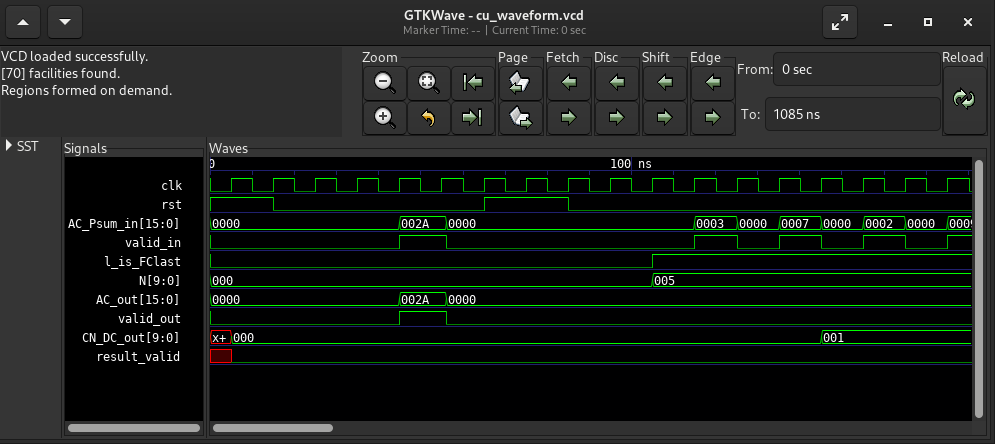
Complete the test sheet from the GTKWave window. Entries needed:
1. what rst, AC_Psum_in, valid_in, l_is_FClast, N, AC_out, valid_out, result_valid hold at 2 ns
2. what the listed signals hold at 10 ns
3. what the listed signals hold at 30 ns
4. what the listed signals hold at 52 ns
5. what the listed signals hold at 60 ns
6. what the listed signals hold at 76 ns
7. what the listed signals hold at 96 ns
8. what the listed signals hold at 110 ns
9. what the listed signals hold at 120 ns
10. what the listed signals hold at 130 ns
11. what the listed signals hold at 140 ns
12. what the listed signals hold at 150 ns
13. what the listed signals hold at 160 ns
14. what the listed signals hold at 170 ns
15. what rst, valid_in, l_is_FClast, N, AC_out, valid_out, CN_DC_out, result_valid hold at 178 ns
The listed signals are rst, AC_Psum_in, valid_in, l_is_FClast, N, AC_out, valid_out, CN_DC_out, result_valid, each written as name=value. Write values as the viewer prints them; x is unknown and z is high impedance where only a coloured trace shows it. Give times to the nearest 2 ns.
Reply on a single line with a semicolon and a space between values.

rst=1, AC_Psum_in=0000, valid_in=0, l_is_FClast=0, N=000, AC_out=0000, valid_out=0, result_valid=x; rst=1, AC_Psum_in=0000, valid_in=0, l_is_FClast=0, N=000, AC_out=0000, valid_out=0, CN_DC_out=000, result_valid=0; rst=0, AC_Psum_in=0000, valid_in=0, l_is_FClast=0, N=000, AC_out=0000, valid_out=0, CN_DC_out=000, result_valid=0; rst=0, AC_Psum_in=002A, valid_in=1, l_is_FClast=0, N=000, AC_out=002A, valid_out=1, CN_DC_out=000, result_valid=0; rst=0, AC_Psum_in=0000, valid_in=0, l_is_FClast=0, N=000, AC_out=0000, valid_out=0, CN_DC_out=000, result_valid=0; rst=1, AC_Psum_in=0000, valid_in=0, l_is_FClast=0, N=000, AC_out=0000, valid_out=0, CN_DC_out=000, result_valid=0; rst=0, AC_Psum_in=0000, valid_in=0, l_is_FClast=0, N=000, AC_out=0000, valid_out=0, CN_DC_out=000, result_valid=0; rst=0, AC_Psum_in=0000, valid_in=0, l_is_FClast=1, N=005, AC_out=0000, valid_out=0, CN_DC_out=000, result_valid=0; rst=0, AC_Psum_in=0003, valid_in=1, l_is_FClast=1, N=005, AC_out=0000, valid_out=0, CN_DC_out=000, result_valid=0; rst=0, AC_Psum_in=0000, valid_in=0, l_is_FClast=1, N=005, AC_out=0000, valid_out=0, CN_DC_out=000, result_valid=0; rst=0, AC_Psum_in=0007, valid_in=1, l_is_FClast=1, N=005, AC_out=0000, valid_out=0, CN_DC_out=000, result_valid=0; rst=0, AC_Psum_in=0000, valid_in=0, l_is_FClast=1, N=005, AC_out=0000, valid_out=0, CN_DC_out=001, result_valid=0; rst=0, AC_Psum_in=0002, valid_in=1, l_is_FClast=1, N=005, AC_out=0000, valid_out=0, CN_DC_out=001, result_valid=0; rst=0, AC_Psum_in=0000, valid_in=0, l_is_FClast=1, N=005, AC_out=0000, valid_out=0, CN_DC_out=001, result_valid=0; rst=0, valid_in=1, l_is_FClast=1, N=005, AC_out=0000, valid_out=0, CN_DC_out=001, result_valid=0
